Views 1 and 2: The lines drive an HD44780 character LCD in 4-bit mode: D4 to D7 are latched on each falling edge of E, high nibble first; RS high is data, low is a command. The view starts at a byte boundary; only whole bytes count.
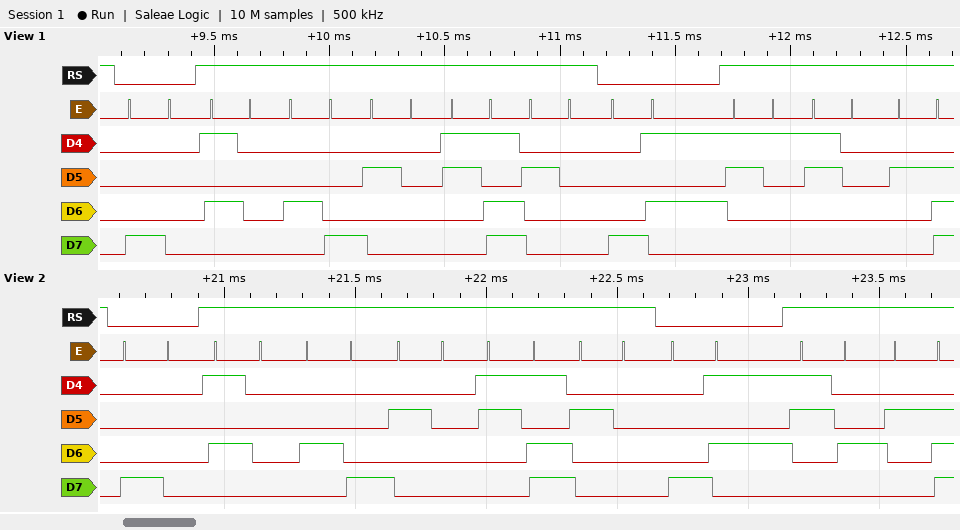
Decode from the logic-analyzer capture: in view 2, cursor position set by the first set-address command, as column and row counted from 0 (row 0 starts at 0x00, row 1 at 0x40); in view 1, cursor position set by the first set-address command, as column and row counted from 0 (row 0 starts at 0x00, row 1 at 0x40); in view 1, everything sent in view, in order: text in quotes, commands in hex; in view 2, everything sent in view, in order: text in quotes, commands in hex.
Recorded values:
column 0, row 0
column 0, row 0
0x80 "PH = " 0x85 "10."
0x80 "PH = " 0x85 "4."
